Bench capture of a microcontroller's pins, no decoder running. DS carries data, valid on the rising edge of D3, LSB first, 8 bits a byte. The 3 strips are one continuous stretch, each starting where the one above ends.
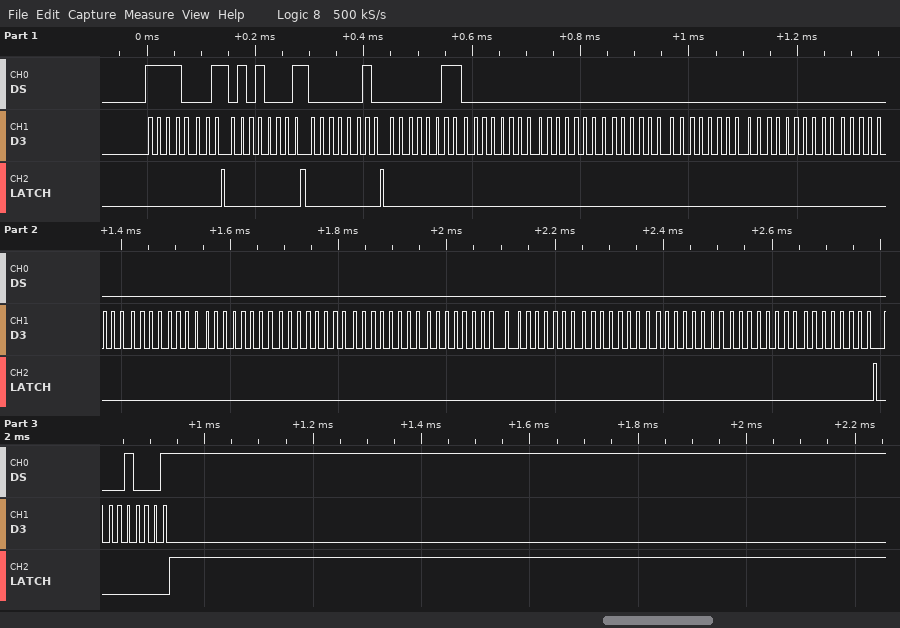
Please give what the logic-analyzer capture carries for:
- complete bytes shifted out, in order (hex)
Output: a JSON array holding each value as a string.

["0x8F 0x8A 0x40 0xC0 0x00 0x00 0x00 0x00 0x00 0x00 0x00 0x00 0x00 0x00 0x00 0x00 0x00 0x00 0x00 0x00 0x88"]
